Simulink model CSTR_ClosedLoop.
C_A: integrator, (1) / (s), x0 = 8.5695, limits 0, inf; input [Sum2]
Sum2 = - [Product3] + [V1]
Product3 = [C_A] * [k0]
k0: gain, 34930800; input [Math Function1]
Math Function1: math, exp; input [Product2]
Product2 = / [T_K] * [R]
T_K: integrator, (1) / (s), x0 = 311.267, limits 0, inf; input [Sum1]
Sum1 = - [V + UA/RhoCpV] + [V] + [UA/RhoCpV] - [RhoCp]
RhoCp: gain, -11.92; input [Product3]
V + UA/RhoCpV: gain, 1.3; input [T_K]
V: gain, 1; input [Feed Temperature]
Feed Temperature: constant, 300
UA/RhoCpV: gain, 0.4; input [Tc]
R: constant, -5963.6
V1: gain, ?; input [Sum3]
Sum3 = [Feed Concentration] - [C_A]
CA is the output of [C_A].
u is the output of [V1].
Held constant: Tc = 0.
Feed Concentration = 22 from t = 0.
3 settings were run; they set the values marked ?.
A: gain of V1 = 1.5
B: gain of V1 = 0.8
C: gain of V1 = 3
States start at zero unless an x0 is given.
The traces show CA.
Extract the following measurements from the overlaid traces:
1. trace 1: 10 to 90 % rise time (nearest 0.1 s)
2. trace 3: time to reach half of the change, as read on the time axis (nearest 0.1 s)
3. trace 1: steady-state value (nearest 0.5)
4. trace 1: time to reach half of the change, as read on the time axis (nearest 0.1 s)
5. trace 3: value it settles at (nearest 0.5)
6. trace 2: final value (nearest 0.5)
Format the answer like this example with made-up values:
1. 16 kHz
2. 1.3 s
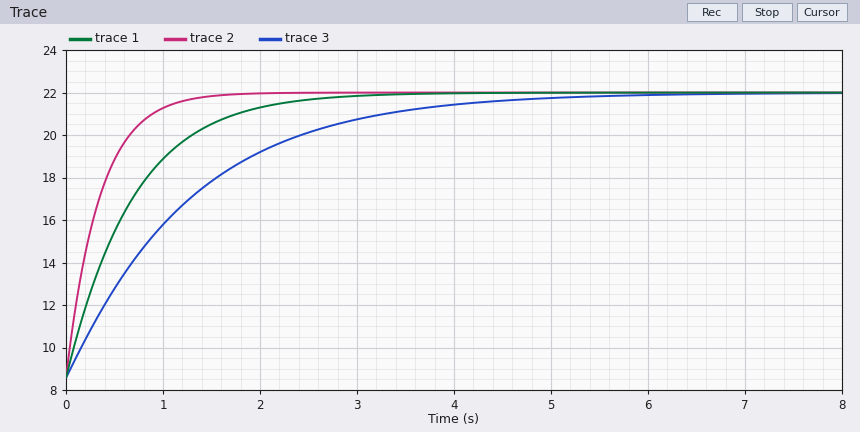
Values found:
1. 1.5 s
2. 0.9 s
3. 22.0
4. 0.5 s
5. 22.0
6. 22.0
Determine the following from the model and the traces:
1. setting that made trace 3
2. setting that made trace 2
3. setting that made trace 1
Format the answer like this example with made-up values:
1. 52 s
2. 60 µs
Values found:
1. B
2. C
3. A
